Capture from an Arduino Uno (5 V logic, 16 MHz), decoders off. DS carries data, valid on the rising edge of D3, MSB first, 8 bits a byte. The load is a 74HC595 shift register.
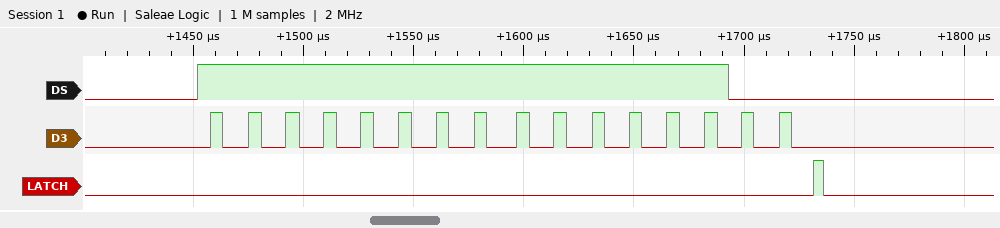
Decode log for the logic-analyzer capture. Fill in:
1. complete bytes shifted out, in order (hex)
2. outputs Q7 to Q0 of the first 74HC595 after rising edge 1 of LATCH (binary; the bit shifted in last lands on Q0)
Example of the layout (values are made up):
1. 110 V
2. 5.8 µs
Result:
1. FF FC
2. 11111100
